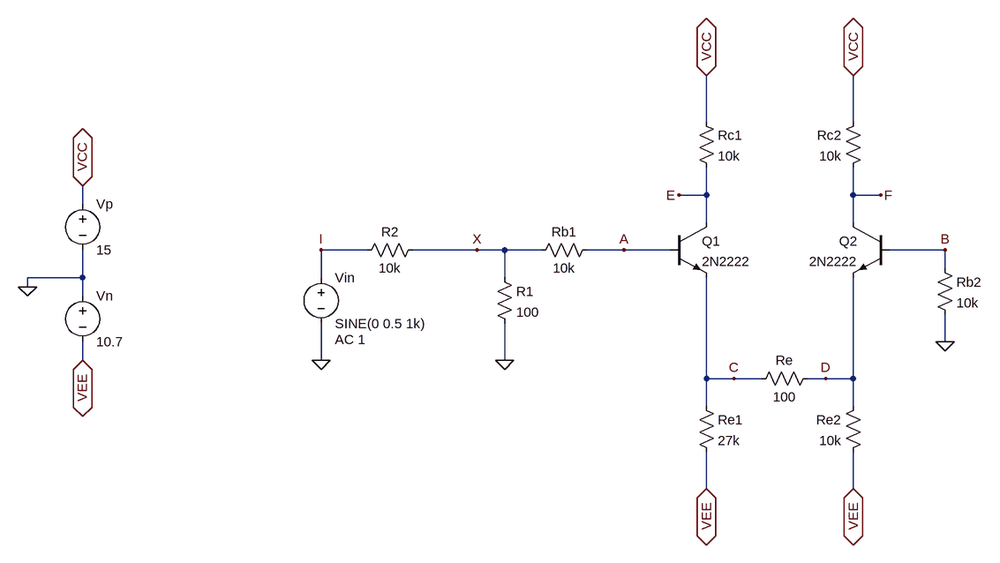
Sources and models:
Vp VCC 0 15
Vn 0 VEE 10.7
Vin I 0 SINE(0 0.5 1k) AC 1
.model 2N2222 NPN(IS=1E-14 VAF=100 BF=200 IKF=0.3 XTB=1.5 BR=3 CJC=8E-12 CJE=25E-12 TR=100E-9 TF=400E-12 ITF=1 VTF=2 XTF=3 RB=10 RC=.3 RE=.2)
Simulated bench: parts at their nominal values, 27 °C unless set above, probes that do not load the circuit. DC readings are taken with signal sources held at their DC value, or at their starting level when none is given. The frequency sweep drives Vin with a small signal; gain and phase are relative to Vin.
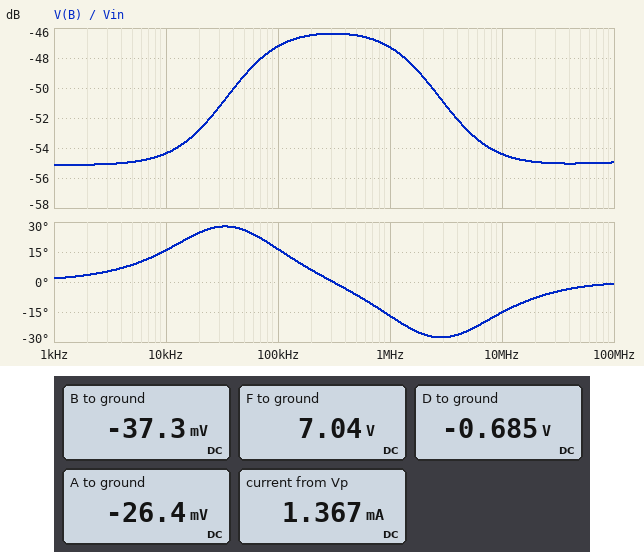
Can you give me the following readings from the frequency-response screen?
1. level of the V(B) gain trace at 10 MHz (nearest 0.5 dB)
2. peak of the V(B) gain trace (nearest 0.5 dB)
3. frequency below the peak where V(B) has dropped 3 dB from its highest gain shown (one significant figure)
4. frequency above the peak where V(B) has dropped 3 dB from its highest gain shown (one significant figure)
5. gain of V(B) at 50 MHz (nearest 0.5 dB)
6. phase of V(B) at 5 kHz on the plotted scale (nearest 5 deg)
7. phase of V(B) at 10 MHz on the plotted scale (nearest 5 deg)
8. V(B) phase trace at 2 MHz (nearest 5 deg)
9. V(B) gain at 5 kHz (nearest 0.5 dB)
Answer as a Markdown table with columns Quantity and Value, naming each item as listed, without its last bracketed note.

| Quantity | Value |
|---|---|
| level of the V(B) gain trace at 10 MHz | -54.5 dB |
| peak of the V(B) gain trace | -46.5 dB |
| frequency below the peak where V(B) has dropped 3 dB from its highest gain shown | 50 kHz |
| frequency above the peak where V(B) has dropped 3 dB from its highest gain shown | 2 MHz |
| gain of V(B) at 50 MHz | -55.0 dB |
| phase of V(B) at 5 kHz on the plotted scale | 10 deg |
| phase of V(B) at 10 MHz on the plotted scale | -15 deg |
| V(B) phase trace at 2 MHz | -25 deg |
| V(B) gain at 5 kHz | -55.0 dB |
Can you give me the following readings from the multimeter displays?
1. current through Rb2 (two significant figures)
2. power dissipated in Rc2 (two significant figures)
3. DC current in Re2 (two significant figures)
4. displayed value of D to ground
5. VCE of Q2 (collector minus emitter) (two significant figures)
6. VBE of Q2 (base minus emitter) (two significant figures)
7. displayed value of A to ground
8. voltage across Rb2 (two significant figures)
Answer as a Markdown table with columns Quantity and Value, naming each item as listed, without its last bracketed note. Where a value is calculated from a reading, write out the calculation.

| Quantity | Value |
|---|---|
| current through Rb2 | (0 V - (-37.3 mV)) / 10 kΩ = 3.7 µA |
| power dissipated in Rc2 | (15 V - 7.04 V)^2 / 10 kΩ = 6.3 mW |
| DC current in Re2 | (-685 mV - (-10.7 V)) / 10 kΩ = 1.0 mA |
| displayed value of D to ground | -0.685 V |
| VCE of Q2 (collector minus emitter) | 7.04 V - (-685 mV) = 7.7 V |
| VBE of Q2 (base minus emitter) | -37.3 mV - (-685 mV) = 650 mV |
| displayed value of A to ground | -26.4 mV |
| voltage across Rb2 | 0 V - (-37.3 mV) = 37 mV |
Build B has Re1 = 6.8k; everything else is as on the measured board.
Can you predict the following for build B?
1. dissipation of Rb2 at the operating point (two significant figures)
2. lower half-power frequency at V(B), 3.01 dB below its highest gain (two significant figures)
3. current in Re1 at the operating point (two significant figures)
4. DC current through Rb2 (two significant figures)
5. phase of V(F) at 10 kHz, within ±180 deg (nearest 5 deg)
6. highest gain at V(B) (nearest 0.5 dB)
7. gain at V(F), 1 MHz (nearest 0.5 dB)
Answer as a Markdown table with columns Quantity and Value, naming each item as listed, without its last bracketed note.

| Quantity | Value |
|---|---|
| dissipation of Rb2 at the operating point | 300 nW |
| lower half-power frequency at V(B), 3.01 dB below its highest gain | 28 kHz |
| current in Re1 at the operating point | 1.5 mA |
| DC current through Rb2 | 5.5 µA |
| phase of V(F) at 10 kHz, within ±180 deg | -15 deg |
| highest gain at V(B) | -47.5 dB |
| gain at V(F), 1 MHz | -38.5 dB |
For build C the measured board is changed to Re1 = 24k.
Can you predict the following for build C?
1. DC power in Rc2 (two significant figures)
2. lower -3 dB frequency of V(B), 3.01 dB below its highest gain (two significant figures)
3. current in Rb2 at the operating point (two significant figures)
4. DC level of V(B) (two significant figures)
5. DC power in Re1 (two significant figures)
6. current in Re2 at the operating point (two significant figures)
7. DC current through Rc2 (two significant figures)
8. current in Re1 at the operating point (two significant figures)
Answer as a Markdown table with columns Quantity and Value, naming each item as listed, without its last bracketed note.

| Quantity | Value |
|---|---|
| DC power in Rc2 | 6.6 mW |
| lower -3 dB frequency of V(B), 3.01 dB below its highest gain | 46 kHz |
| current in Rb2 at the operating point | 3.8 µA |
| DC level of V(B) | -38 mV |
| DC power in Re1 | 4.2 mW |
| current in Re2 at the operating point | 1.0 mA |
| DC current through Rc2 | 810 µA |
| current in Re1 at the operating point | 420 µA |
